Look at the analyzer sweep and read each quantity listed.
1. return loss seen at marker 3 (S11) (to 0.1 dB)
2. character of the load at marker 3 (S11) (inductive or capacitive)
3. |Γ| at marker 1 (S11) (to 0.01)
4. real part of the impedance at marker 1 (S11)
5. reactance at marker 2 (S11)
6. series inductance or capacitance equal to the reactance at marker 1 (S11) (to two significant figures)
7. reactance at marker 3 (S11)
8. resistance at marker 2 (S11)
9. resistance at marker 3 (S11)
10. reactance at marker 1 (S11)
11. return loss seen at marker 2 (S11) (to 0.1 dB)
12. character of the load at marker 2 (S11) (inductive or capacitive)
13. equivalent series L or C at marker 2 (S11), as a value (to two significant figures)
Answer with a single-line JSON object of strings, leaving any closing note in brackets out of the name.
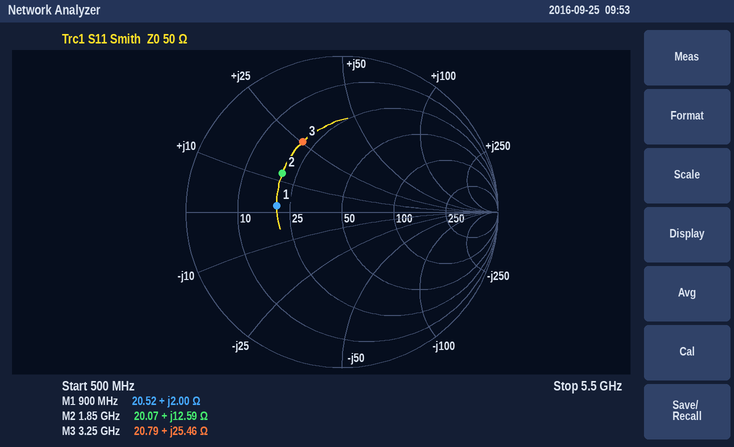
{"return loss seen at marker 3 (S11)": "5.8 dB", "character of the load at marker 3 (S11)": "inductive", "|Γ| at marker 1 (S11)": "0.42", "real part of the impedance at marker 1": "20.52 Ω", "reactance at marker 2": "+12.59 Ω", "series inductance or capacitance equal to the reactance at marker 1 (S11)": "350 pH", "reactance at marker 3": "+25.46 Ω", "resistance at marker 2": "20.07 Ω", "resistance at marker 3": "20.79 Ω", "reactance at marker 1": "+2.00 Ω", "return loss seen at marker 2 (S11)": "6.8 dB", "character of the load at marker 2 (S11)": "inductive", "equivalent series L or C at marker 2 (S11), as a value": "1.1 nH"}
